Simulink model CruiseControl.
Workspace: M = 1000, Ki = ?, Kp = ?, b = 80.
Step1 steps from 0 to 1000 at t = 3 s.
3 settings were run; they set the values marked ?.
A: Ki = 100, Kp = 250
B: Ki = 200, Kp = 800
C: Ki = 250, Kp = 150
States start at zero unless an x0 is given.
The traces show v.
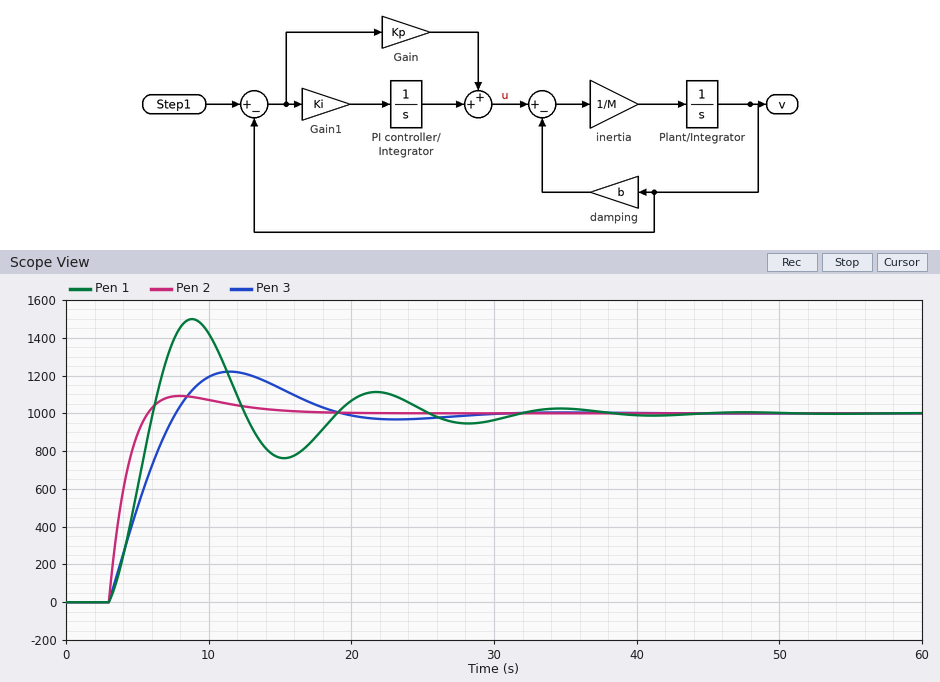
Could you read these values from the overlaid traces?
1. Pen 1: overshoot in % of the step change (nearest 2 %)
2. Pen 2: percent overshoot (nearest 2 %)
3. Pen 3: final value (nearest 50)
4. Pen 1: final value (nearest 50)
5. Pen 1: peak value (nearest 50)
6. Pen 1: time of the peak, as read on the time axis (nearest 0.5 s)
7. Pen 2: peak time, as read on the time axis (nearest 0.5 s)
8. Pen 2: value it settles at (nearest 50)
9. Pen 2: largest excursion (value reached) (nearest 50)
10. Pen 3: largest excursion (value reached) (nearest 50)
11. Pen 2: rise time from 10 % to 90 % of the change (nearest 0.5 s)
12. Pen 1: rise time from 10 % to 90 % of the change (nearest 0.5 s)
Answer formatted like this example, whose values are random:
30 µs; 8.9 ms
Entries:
50 %; 10 %; 1000; 1000; 1500; 9.0 s; 8.0 s; 1000; 1100; 1200; 2.0 s; 2.5 s
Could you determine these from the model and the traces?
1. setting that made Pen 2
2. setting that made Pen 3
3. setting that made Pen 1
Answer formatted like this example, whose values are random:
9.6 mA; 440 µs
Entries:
B; A; C
